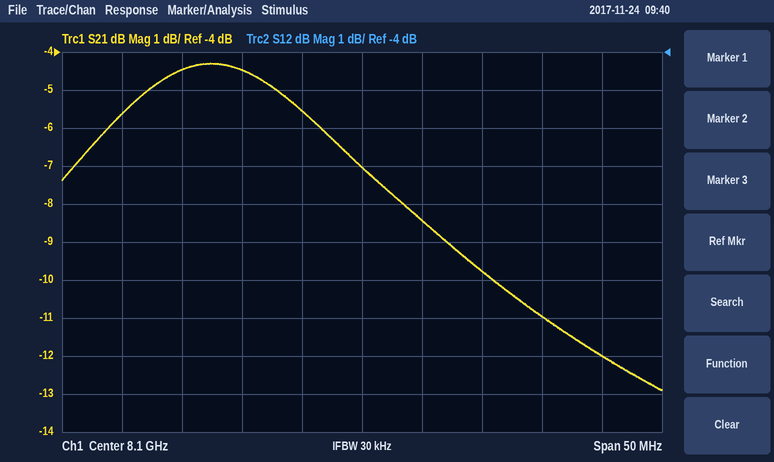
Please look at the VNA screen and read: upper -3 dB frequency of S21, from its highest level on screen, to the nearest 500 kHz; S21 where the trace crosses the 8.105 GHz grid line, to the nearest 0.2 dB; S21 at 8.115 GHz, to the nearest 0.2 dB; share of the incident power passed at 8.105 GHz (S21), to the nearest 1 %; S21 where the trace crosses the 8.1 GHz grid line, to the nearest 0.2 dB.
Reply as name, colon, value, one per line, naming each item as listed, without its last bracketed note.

upper -3 dB frequency of S21, from its highest level on screen, to the nearest 500 kHz: 8.1010 GHz
S21 where the trace crosses the 8.105 GHz grid line, to the nearest 0.2 dB: -8.4 dB
S21 at 8.115 GHz, to the nearest 0.2 dB: -11.0 dB
share of the incident power passed at 8.105 GHz (S21), to the nearest 1 %: 14 %
S21 where the trace crosses the 8.1 GHz grid line, to the nearest 0.2 dB: -7.0 dB
